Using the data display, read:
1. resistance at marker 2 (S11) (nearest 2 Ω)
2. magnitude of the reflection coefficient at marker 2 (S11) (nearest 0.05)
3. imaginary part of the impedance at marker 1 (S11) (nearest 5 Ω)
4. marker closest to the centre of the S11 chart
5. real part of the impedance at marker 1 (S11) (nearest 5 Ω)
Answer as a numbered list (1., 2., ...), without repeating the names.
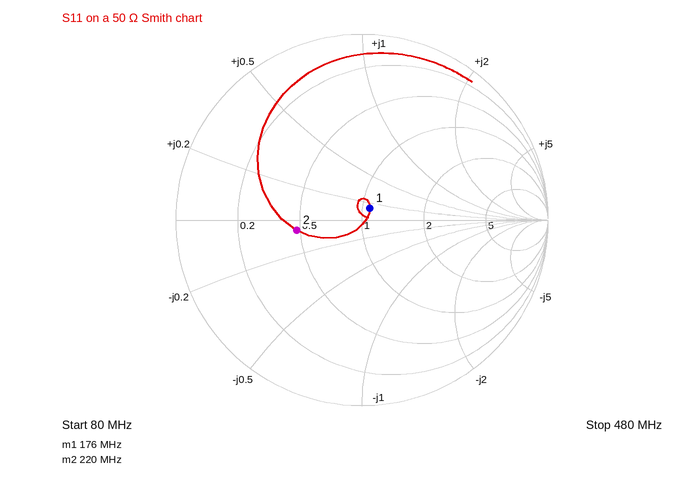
1. 24 Ω
2. 0.35
3. +5 Ω
4. marker 1
5. 55 Ω
